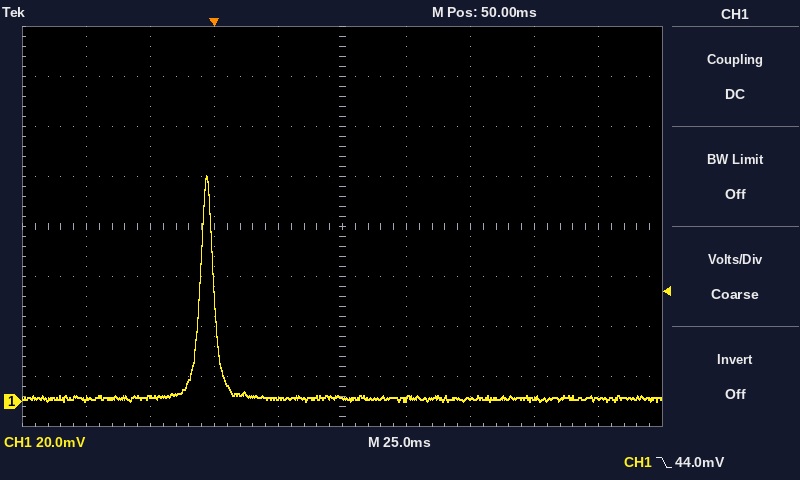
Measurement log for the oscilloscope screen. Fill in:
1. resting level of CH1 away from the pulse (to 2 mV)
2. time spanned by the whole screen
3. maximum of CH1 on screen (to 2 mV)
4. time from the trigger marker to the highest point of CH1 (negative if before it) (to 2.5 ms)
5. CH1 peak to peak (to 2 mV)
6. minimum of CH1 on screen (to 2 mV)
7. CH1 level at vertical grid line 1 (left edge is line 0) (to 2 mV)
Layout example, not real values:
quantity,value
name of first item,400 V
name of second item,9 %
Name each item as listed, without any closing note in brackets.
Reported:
quantity,value
resting level of CH1 away from the pulse,2 mV
time spanned by the whole screen,250 ms
maximum of CH1 on screen,90 mV
time from the trigger marker to the highest point of CH1 (negative if before it),-2.5 ms
CH1 peak to peak,90 mV
minimum of CH1 on screen,0 mV
CH1 level at vertical grid line 1 (left edge is line 0),2 mV
